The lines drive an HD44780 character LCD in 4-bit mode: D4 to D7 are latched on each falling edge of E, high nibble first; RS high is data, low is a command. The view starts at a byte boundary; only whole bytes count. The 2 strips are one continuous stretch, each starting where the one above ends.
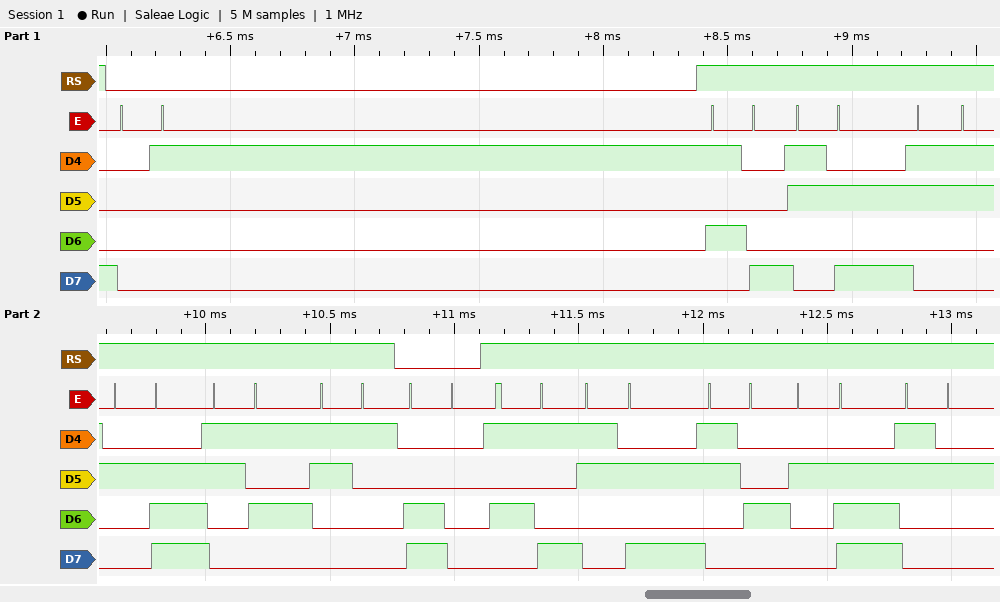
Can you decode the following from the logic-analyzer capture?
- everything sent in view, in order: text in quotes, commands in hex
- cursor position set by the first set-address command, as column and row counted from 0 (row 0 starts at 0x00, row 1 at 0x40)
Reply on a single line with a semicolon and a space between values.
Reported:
0x01 "X:3.51" 0xC0 "Y:4.2"; column 0, row 1
